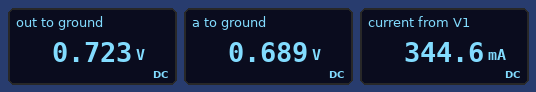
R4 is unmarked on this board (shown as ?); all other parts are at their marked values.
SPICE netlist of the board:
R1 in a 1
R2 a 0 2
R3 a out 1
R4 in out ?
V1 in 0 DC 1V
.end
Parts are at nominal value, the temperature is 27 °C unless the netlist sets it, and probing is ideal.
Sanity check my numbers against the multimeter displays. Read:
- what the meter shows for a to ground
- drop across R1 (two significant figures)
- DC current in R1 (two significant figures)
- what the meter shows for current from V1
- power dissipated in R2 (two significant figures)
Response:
0.689 V
310 mV
310 mA
344.6 mA
240 mW
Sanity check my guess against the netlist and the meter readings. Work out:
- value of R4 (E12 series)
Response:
8.2 Ω
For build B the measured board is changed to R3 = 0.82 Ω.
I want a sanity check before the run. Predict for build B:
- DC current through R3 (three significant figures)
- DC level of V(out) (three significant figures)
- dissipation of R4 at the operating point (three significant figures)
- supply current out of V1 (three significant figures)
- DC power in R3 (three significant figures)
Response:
34.4 mA
718 mV
9.71 mW
345 mA
971 µW
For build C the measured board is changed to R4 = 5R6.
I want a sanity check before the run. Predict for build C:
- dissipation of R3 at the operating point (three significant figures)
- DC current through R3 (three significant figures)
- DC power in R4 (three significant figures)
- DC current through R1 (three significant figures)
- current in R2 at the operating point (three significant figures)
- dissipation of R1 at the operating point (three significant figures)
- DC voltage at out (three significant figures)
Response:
2.10 mW
45.9 mA
11.8 mW
303 mA
349 mA
91.7 mW
743 mV
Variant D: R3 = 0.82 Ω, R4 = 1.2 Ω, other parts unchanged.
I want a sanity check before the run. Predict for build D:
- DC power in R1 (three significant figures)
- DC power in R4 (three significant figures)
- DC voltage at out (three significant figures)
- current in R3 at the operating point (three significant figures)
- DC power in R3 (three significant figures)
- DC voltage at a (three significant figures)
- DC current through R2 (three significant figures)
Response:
62.8 mW
18.5 mW
851 mV
124 mA
12.6 mW
749 mV
375 mA
